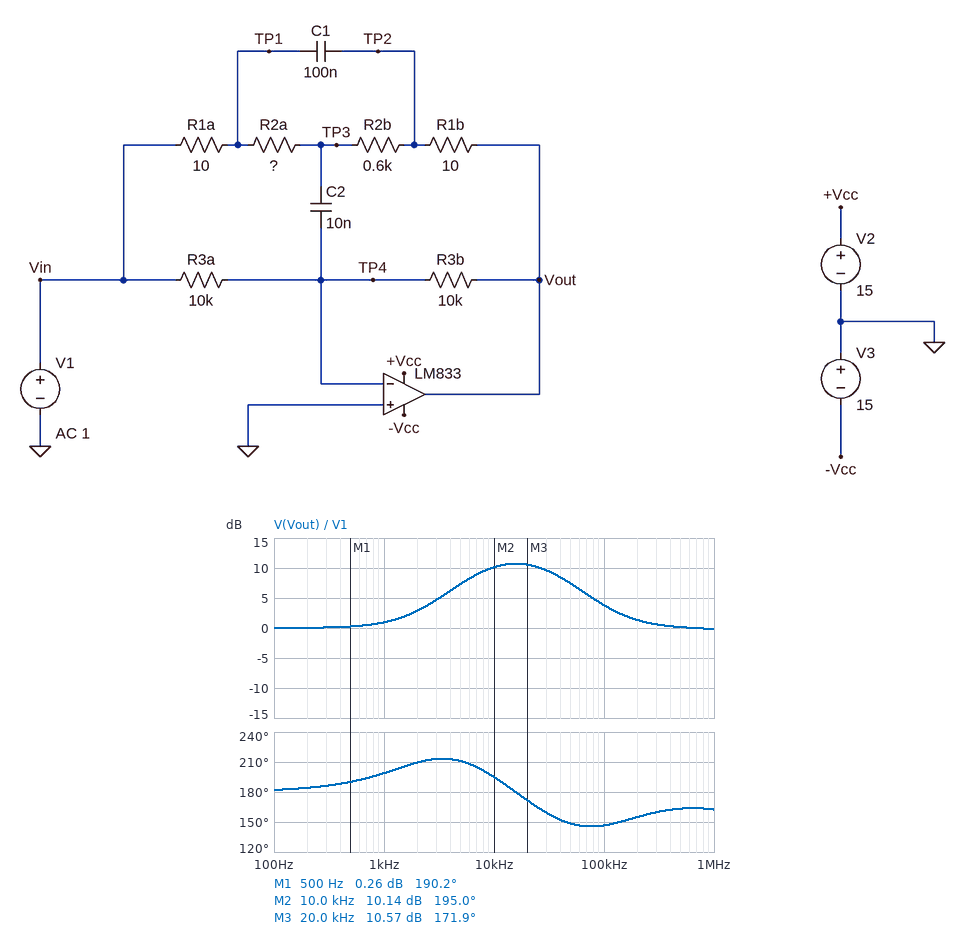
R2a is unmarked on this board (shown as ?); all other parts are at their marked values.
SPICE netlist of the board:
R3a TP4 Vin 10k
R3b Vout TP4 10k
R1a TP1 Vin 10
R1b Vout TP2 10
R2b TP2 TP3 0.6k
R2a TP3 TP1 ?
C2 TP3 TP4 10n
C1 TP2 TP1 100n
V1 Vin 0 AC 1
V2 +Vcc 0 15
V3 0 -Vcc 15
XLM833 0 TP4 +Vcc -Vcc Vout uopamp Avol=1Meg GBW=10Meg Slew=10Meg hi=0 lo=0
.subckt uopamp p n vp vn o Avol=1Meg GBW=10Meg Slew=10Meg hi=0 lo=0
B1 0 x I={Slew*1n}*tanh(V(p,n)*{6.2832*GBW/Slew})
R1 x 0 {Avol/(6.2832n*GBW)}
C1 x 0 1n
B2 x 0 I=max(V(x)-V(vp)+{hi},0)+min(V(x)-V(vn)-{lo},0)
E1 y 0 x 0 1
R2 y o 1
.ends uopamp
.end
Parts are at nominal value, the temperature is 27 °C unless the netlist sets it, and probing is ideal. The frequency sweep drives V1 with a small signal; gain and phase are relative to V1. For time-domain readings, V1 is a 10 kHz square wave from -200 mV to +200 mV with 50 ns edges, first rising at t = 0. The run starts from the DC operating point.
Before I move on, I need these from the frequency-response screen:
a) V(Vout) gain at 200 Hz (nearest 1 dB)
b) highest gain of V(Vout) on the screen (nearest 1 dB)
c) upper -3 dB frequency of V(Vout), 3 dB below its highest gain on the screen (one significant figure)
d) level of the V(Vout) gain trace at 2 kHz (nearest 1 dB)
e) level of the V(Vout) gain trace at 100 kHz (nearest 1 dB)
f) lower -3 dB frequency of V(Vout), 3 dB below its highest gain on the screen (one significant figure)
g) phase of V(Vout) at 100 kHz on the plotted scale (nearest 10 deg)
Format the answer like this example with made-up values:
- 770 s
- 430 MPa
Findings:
- 0 dB
- 11 dB
- 50 kHz
- 3 dB
- 4 dB
- 5 kHz
- 150 deg
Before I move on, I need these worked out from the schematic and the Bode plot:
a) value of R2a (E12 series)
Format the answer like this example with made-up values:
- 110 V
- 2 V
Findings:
- 150 Ω
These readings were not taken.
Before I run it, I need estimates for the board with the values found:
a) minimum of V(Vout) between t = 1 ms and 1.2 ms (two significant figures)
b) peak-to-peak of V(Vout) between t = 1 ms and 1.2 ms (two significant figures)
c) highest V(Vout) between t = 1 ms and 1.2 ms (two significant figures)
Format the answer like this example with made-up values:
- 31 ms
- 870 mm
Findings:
- -890 mV
- 1.8 V
- 890 mV
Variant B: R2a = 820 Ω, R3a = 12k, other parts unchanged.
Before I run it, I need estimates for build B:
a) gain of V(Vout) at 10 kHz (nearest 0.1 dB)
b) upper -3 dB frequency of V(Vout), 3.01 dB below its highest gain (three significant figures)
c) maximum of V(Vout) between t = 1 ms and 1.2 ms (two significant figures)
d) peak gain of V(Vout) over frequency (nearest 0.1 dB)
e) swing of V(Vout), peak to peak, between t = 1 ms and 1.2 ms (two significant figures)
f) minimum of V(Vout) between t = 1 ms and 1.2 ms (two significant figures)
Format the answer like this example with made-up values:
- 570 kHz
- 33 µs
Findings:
- -2.6 dB
- 4.91 MHz
- 230 mV
- -0.2 dB
- 470 mV
- -230 mV
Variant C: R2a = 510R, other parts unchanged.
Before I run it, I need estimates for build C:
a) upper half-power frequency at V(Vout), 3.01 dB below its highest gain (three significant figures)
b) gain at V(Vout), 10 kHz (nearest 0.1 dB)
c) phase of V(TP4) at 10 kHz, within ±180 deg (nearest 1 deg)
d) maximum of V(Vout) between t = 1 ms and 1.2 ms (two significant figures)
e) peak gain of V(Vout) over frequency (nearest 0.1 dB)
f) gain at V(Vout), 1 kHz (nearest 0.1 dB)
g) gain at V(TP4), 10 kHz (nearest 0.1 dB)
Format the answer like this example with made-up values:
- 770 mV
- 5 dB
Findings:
- 3.36 MHz
- 1.2 dB
- 92 deg
- 240 mV
- 1.3 dB
- 0.1 dB
- -58.7 dB
